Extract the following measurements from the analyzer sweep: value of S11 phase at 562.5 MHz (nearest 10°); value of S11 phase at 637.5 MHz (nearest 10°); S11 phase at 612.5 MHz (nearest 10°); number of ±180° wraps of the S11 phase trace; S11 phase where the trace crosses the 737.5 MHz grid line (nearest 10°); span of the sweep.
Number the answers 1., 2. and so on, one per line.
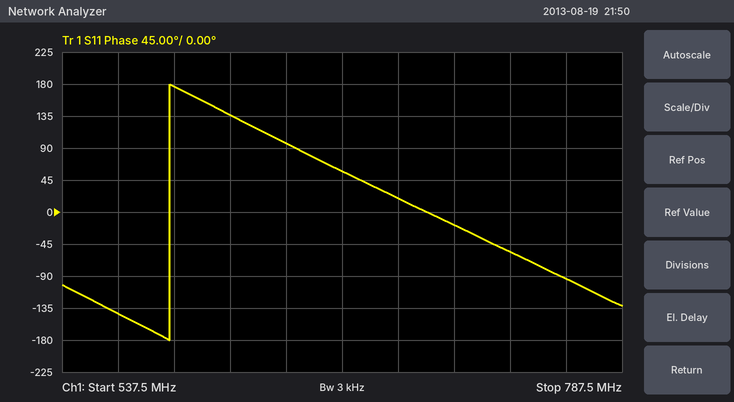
1. -140°
2. 100°
3. 140°
4. 1
5. -60°
6. 250 MHz
